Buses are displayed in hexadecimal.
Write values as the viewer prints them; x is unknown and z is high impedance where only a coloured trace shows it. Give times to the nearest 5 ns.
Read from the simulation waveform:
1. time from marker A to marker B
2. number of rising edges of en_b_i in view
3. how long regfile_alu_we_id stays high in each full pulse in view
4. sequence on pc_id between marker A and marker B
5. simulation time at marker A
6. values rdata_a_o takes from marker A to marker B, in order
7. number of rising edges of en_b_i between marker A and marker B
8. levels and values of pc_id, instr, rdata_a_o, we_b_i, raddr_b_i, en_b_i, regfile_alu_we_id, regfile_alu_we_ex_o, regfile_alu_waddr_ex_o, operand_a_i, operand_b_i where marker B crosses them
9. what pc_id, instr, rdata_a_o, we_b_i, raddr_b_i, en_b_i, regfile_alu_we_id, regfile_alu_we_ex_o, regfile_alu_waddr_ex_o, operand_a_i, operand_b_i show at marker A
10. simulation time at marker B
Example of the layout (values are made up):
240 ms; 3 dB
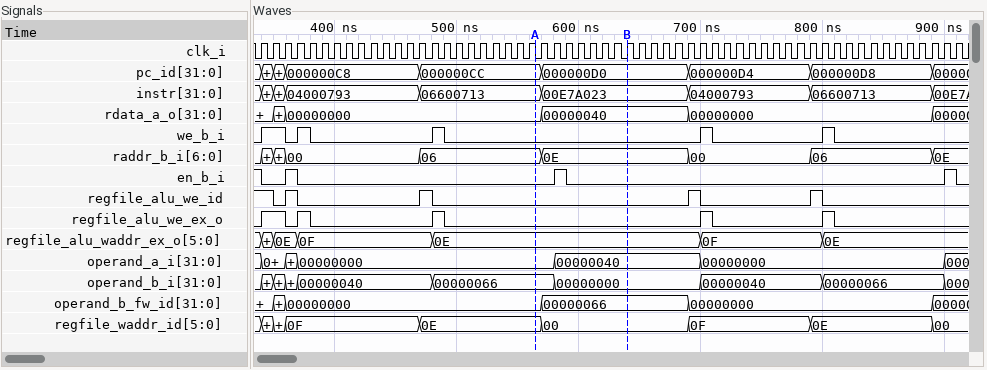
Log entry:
75 ns; 3; 10 ns, 10 ns, 10 ns, 10 ns; 000000CC, 000000D0; 565 ns; 00000000, 00000040; 1; pc_id=000000D0, instr=00E7A023, rdata_a_o=00000040, we_b_i=0, raddr_b_i=0E, en_b_i=0, regfile_alu_we_id=0, regfile_alu_we_ex_o=0, regfile_alu_waddr_ex_o=0E, operand_a_i=00000040, operand_b_i=00000000; pc_id=000000CC, instr=06600713, rdata_a_o=00000000, we_b_i=0, raddr_b_i=06, en_b_i=0, regfile_alu_we_id=0, regfile_alu_we_ex_o=0, regfile_alu_waddr_ex_o=0E, operand_a_i=00000000, operand_b_i=00000066; 640 ns
